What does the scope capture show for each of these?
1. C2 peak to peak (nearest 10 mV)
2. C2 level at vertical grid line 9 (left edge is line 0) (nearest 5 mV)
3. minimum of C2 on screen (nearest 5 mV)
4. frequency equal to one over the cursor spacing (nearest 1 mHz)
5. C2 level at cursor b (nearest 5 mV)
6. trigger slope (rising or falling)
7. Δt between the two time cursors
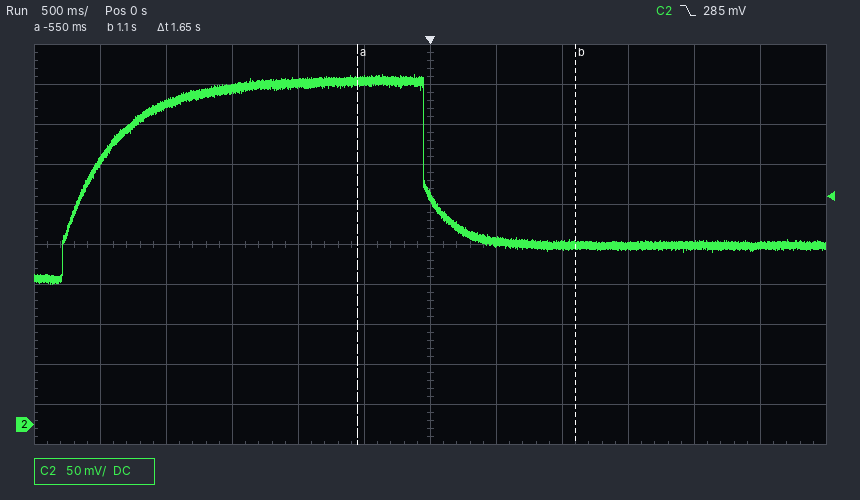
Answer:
260 mV
225 mV
175 mV
606 mHz
225 mV
falling
1.65 s
